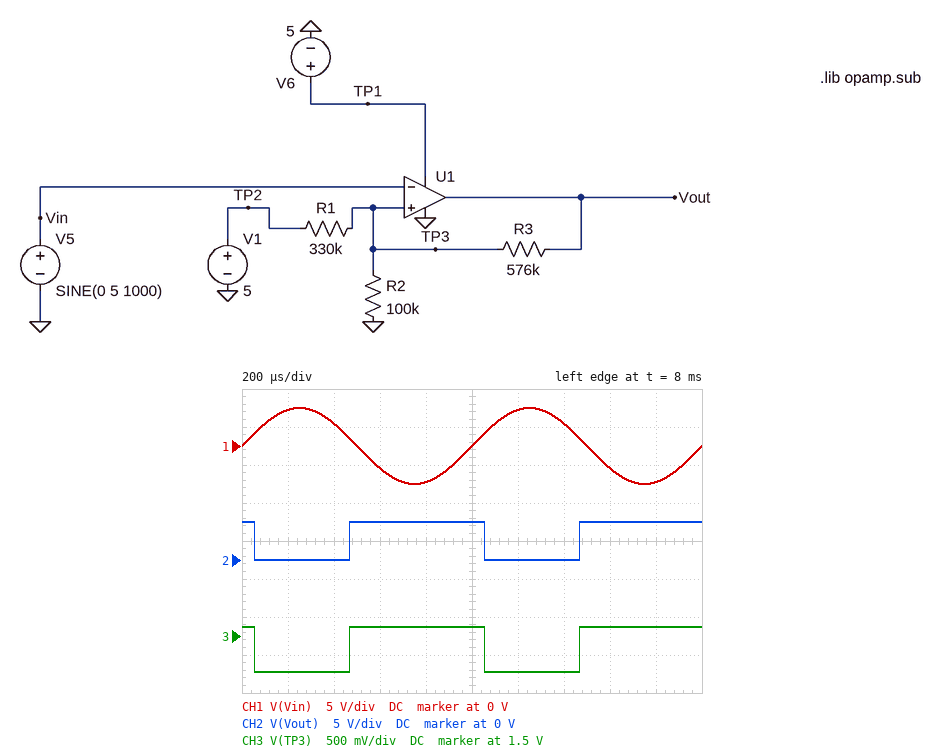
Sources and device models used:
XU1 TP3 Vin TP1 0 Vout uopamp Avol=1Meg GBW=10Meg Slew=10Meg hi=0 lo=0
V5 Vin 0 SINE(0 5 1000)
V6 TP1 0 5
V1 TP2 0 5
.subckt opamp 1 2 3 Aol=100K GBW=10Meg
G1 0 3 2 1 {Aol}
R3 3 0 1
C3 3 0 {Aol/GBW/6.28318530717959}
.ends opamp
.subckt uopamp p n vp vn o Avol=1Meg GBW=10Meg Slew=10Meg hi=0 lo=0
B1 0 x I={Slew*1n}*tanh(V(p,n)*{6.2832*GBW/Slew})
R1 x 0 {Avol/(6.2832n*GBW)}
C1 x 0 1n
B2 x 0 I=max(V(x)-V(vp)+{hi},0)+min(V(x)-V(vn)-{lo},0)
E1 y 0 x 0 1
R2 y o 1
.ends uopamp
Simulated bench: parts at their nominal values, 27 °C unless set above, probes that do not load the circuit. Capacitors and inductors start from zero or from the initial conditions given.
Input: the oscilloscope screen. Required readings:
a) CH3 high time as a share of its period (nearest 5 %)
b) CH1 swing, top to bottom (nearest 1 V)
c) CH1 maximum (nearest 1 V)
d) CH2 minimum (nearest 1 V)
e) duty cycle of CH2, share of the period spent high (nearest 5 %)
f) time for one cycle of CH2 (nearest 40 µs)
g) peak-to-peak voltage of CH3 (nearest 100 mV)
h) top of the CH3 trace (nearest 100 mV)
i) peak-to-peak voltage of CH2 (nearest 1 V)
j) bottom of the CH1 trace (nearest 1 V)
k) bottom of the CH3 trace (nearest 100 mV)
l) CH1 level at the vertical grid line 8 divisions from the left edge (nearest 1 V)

60 %
10 V
5 V
0 V
60 %
1.00 ms
600 mV
1.6 V
5 V
-5 V
1.0 V
-3 V
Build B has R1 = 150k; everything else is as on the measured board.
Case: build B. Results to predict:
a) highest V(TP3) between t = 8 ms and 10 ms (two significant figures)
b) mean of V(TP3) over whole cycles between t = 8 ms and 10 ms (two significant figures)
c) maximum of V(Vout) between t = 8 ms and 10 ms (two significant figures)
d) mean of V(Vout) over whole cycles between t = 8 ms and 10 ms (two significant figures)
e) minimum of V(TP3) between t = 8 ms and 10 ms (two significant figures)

2.3 V
2.1 V
5.0 V
3.2 V
1.8 V
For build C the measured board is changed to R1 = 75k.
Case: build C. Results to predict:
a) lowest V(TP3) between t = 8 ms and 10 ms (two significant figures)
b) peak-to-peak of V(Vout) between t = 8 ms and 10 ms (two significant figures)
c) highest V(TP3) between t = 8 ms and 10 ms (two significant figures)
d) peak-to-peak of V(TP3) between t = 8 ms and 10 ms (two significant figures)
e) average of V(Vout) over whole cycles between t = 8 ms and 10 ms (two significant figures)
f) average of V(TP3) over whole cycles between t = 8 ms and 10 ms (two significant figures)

2.7 V
5.0 V
3.0 V
350 mV
3.5 V
2.9 V
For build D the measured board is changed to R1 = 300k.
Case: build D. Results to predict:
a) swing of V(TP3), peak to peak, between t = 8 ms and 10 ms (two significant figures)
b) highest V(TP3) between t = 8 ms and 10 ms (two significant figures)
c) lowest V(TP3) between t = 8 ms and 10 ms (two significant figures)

580 mV
1.7 V
1.1 V
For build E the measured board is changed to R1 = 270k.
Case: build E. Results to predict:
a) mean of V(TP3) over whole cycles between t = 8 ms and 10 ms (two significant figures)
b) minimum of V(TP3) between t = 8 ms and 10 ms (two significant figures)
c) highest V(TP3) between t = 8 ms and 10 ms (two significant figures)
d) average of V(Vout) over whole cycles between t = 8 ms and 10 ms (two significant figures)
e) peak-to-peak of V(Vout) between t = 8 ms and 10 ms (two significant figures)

1.5 V
1.2 V
1.8 V
3.0 V
5.0 V
